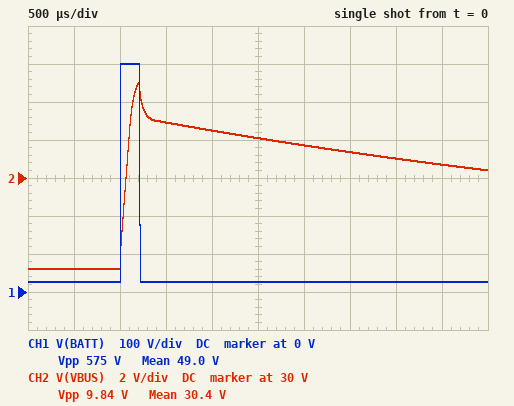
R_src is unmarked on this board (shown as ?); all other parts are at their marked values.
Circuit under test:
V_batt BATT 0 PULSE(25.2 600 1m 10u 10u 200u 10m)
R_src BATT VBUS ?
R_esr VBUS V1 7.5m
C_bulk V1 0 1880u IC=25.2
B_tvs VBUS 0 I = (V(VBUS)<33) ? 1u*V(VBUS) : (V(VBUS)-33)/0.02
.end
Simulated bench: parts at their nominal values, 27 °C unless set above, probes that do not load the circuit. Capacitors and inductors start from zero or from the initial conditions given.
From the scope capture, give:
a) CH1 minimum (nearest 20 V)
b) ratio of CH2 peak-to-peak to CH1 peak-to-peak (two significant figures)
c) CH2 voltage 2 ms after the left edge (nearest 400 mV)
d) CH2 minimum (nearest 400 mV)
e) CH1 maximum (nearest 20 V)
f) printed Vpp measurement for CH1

20 V
0.017
32.4 V
25.2 V
600 V
575 V
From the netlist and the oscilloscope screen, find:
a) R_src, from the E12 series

4.7 Ω
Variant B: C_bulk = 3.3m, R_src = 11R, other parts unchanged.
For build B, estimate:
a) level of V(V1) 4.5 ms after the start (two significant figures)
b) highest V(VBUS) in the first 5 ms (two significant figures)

28 V
29 V
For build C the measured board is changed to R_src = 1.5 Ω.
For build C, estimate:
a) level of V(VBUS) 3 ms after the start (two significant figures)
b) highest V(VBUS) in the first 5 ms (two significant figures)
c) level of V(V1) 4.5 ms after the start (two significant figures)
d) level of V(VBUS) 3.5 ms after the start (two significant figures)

30 V
40 V
28 V
29 V
